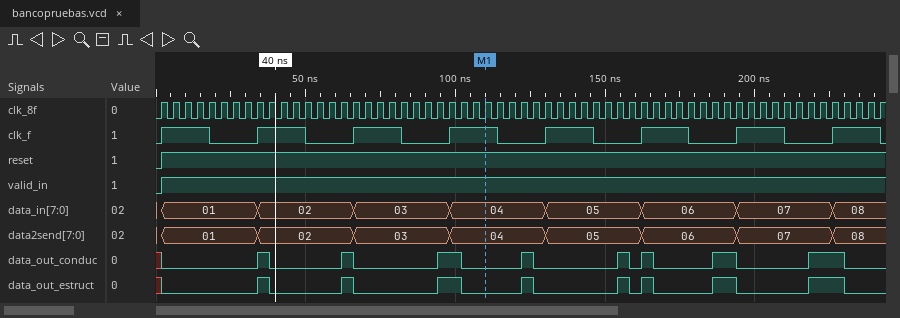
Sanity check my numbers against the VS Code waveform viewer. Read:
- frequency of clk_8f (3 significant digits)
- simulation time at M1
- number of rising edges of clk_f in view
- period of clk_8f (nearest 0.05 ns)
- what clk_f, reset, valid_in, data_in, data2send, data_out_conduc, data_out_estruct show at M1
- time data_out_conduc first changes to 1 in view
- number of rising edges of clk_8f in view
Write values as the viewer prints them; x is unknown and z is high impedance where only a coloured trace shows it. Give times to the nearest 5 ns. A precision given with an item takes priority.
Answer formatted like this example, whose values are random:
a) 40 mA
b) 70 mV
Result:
a) 250 MHz
b) 110 ns
c) 8
d) 4 ns
e) clk_f=1, reset=1, valid_in=1, data_in=04, data2send=04, data_out_conduc=0, data_out_estruct=0
f) 35 ns
g) 61
